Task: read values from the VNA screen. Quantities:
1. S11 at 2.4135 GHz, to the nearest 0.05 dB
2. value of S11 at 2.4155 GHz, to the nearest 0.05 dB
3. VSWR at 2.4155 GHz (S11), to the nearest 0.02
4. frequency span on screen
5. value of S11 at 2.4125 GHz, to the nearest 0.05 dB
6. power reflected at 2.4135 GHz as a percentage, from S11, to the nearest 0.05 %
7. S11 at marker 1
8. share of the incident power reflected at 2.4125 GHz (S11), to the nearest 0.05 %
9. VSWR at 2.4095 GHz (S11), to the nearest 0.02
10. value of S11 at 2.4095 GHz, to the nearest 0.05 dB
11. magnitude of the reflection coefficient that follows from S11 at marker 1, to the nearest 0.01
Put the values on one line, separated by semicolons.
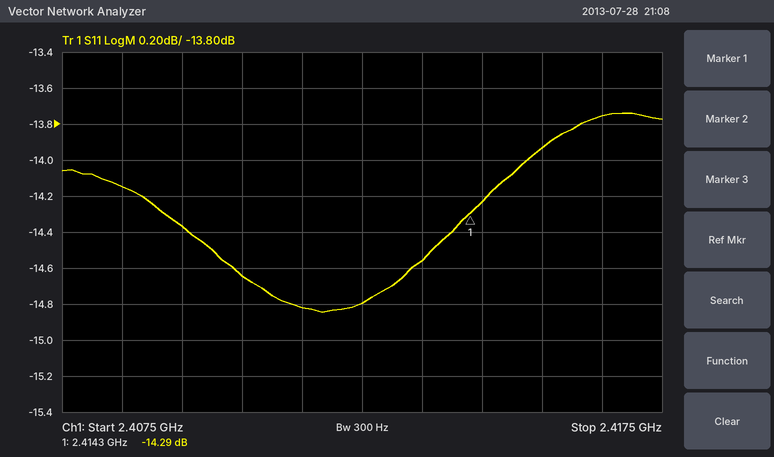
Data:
-14.55 dB; -13.95 dB; 1.50; 10 MHz; -14.80 dB; 3.50 %; -14.29 dB; 3.30 %; 1.48; -14.35 dB; 0.19
